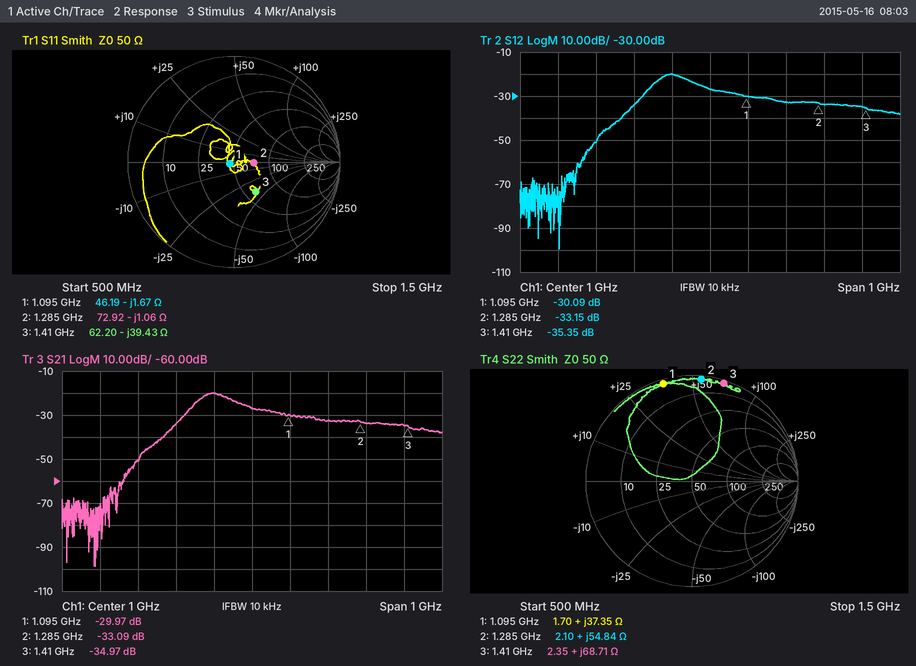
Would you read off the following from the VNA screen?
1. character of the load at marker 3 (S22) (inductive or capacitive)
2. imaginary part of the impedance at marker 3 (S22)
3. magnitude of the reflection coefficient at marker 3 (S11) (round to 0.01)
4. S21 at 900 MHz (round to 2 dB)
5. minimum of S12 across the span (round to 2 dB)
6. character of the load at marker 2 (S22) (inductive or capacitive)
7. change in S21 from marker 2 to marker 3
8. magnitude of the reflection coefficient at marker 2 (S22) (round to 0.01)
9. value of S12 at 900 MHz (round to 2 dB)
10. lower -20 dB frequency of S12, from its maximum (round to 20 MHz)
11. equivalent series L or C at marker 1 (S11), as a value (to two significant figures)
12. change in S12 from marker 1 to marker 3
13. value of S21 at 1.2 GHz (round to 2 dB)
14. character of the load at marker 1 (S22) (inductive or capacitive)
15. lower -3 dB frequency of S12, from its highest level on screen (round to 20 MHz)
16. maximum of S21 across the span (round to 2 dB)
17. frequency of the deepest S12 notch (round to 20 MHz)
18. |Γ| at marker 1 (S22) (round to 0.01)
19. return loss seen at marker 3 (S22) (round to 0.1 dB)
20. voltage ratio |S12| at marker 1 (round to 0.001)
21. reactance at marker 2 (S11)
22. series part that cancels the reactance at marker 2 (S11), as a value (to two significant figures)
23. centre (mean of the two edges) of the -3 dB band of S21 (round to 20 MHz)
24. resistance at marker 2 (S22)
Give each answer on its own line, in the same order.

inductive
+68.71 Ω
0.35
-20 dB
-100 dB
inductive
-1.88 dB
0.96
-20 dB
760 MHz
87 pF
-5.26 dB
-32 dB
inductive
860 MHz
-20 dB
600 MHz
0.96
0.3 dB
0.031
-1.06 Ω
130 pH
900 MHz
2.10 Ω
